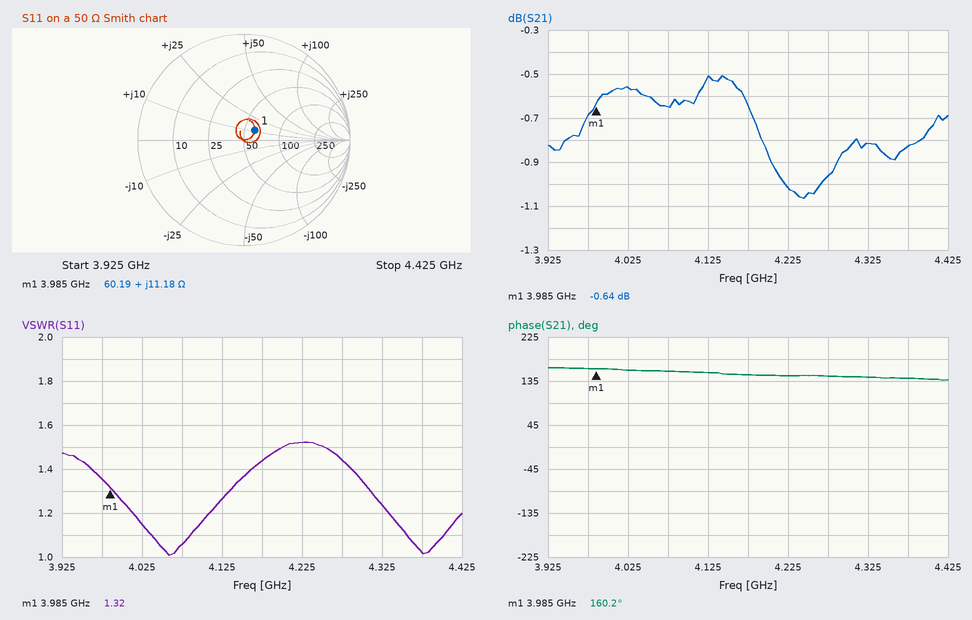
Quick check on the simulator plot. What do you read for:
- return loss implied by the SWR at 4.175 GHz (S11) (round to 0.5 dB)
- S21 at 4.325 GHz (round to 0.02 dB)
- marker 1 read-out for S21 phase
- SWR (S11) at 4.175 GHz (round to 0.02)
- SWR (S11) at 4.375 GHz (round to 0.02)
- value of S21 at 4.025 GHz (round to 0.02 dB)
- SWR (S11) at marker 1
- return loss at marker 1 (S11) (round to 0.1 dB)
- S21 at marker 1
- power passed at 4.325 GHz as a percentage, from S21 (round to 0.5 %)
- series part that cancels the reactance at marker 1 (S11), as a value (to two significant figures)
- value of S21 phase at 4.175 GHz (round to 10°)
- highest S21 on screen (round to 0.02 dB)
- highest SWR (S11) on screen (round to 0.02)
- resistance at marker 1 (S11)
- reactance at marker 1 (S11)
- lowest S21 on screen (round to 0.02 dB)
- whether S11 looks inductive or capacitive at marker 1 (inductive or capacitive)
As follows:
15.0 dB
-0.82 dB
160.2°
1.44
1.02
-0.56 dB
1.32
17.3 dB
-0.64 dB
83.0 %
3.6 pF
150°
-0.50 dB
1.52
60.19 Ω
+11.18 Ω
-1.06 dB
inductive
